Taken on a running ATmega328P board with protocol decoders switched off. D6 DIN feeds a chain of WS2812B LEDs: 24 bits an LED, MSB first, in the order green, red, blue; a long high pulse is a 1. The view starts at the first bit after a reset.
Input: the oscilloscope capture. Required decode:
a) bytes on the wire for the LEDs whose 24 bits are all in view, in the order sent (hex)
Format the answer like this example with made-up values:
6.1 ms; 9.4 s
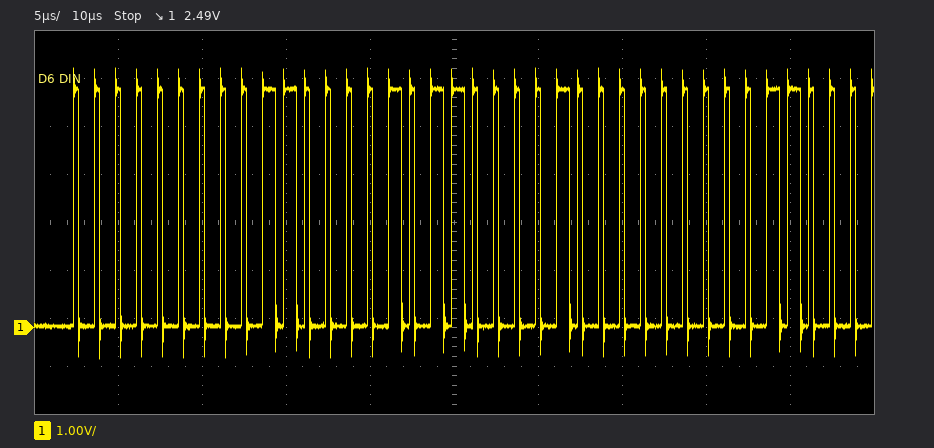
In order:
00 61 61
